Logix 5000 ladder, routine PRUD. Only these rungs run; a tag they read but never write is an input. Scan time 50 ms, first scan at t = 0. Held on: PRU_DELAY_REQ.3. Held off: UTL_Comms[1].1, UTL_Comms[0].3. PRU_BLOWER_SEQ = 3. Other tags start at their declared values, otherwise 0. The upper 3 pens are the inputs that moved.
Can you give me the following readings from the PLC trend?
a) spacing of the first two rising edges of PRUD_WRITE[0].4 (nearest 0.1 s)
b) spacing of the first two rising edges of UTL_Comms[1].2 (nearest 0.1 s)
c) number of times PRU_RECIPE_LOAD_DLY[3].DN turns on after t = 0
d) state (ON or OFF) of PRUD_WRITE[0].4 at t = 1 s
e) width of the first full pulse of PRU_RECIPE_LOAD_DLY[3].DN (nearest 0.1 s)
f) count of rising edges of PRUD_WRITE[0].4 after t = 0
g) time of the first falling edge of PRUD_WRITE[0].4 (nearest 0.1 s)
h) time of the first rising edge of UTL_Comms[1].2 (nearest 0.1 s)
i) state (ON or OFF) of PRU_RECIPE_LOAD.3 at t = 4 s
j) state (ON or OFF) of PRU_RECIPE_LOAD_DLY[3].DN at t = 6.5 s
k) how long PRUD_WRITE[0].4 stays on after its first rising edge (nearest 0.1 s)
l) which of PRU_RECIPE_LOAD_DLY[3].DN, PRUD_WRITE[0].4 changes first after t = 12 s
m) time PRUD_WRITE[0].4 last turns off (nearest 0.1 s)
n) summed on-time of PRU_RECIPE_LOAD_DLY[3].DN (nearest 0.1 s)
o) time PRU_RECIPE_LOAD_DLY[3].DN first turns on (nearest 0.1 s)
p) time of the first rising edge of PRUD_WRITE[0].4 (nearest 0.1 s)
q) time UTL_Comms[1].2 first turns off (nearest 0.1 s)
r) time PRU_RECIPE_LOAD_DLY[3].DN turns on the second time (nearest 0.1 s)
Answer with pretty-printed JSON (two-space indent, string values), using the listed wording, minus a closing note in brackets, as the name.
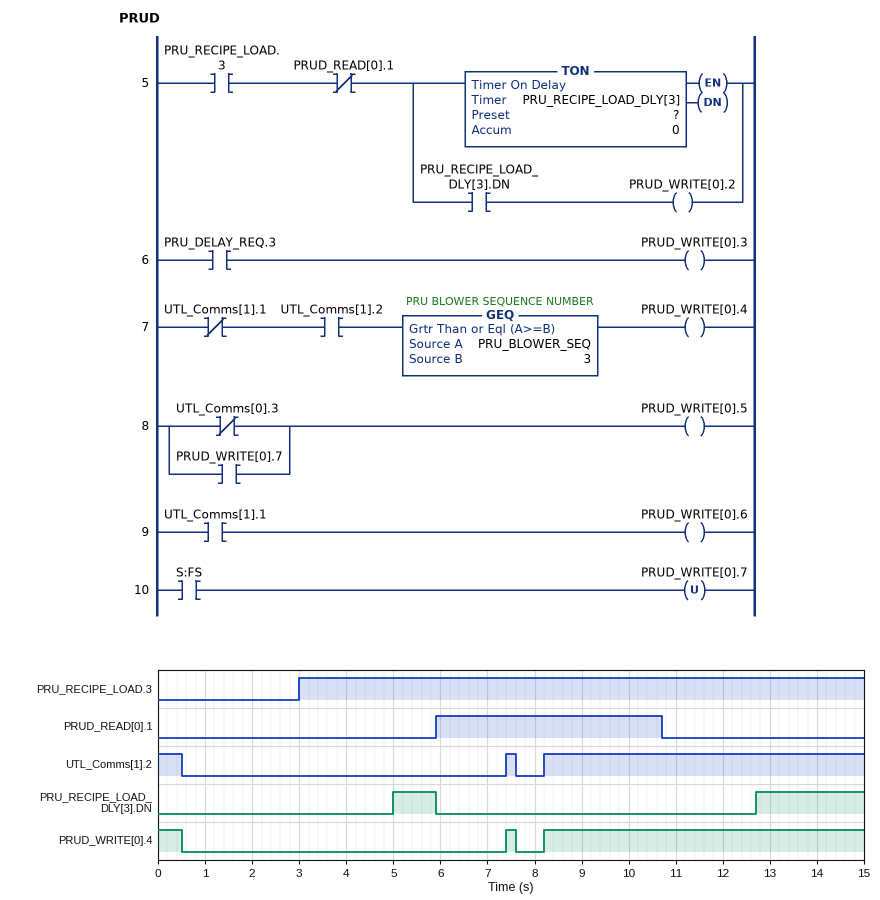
{
  "spacing of the first two rising edges of PRUD_WRITE[0].4": "0.8 s",
  "spacing of the first two rising edges of UTL_Comms[1].2": "0.8 s",
  "number of times PRU_RECIPE_LOAD_DLY[3].DN turns on after t = 0": "2",
  "state (ON or OFF) of PRUD_WRITE[0].4 at t = 1 s": "OFF",
  "width of the first full pulse of PRU_RECIPE_LOAD_DLY[3].DN": "0.9 s",
  "count of rising edges of PRUD_WRITE[0].4 after t = 0": "2",
  "time of the first falling edge of PRUD_WRITE[0].4": "0.5 s",
  "time of the first rising edge of UTL_Comms[1].2": "7.4 s",
  "state (ON or OFF) of PRU_RECIPE_LOAD.3 at t = 4 s": "ON",
  "state (ON or OFF) of PRU_RECIPE_LOAD_DLY[3].DN at t = 6.5 s": "OFF",
  "how long PRUD_WRITE[0].4 stays on after its first rising edge": "0.2 s",
  "which of PRU_RECIPE_LOAD_DLY[3].DN, PRUD_WRITE[0].4 changes first after t = 12 s": "PRU_RECIPE_LOAD_DLY[3].DN",
  "time PRUD_WRITE[0].4 last turns off": "7.6 s",
  "summed on-time of PRU_RECIPE_LOAD_DLY[3].DN": "3.2 s",
  "time PRU_RECIPE_LOAD_DLY[3].DN first turns on": "5.0 s",
  "time of the first rising edge of PRUD_WRITE[0].4": "7.4 s",
  "time UTL_Comms[1].2 first turns off": "0.5 s",
  "time PRU_RECIPE_LOAD_DLY[3].DN turns on the second time": "12.7 s"
}
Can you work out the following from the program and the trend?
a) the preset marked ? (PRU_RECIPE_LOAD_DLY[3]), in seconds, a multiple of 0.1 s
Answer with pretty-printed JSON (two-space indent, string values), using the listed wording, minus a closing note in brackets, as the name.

{
  "the preset marked ? (PRU_RECIPE_LOAD_DLY[3]), in seconds, a multiple of 0.1 s": "2.0 s"
}
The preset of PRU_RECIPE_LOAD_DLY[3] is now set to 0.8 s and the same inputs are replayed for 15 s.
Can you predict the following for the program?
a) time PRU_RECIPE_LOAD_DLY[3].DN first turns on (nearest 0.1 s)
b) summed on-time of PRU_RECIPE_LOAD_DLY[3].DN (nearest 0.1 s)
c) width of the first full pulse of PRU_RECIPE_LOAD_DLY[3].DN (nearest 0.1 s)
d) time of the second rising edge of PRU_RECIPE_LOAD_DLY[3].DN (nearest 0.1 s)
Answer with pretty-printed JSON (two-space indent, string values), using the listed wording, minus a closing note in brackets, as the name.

{
  "time PRU_RECIPE_LOAD_DLY[3].DN first turns on": "3.8 s",
  "summed on-time of PRU_RECIPE_LOAD_DLY[3].DN": "5.6 s",
  "width of the first full pulse of PRU_RECIPE_LOAD_DLY[3].DN": "2.1 s",
  "time of the second rising edge of PRU_RECIPE_LOAD_DLY[3].DN": "11.5 s"
}
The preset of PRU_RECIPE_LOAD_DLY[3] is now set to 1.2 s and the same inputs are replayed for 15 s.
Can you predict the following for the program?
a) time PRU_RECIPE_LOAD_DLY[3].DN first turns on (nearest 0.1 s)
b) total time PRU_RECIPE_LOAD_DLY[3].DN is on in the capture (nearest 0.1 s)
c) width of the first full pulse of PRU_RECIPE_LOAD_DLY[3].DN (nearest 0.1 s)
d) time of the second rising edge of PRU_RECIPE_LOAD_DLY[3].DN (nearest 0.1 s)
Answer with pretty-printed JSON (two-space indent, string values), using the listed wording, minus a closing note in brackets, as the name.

{
  "time PRU_RECIPE_LOAD_DLY[3].DN first turns on": "4.2 s",
  "total time PRU_RECIPE_LOAD_DLY[3].DN is on in the capture": "4.8 s",
  "width of the first full pulse of PRU_RECIPE_LOAD_DLY[3].DN": "1.7 s",
  "time of the second rising edge of PRU_RECIPE_LOAD_DLY[3].DN": "11.9 s"
}
